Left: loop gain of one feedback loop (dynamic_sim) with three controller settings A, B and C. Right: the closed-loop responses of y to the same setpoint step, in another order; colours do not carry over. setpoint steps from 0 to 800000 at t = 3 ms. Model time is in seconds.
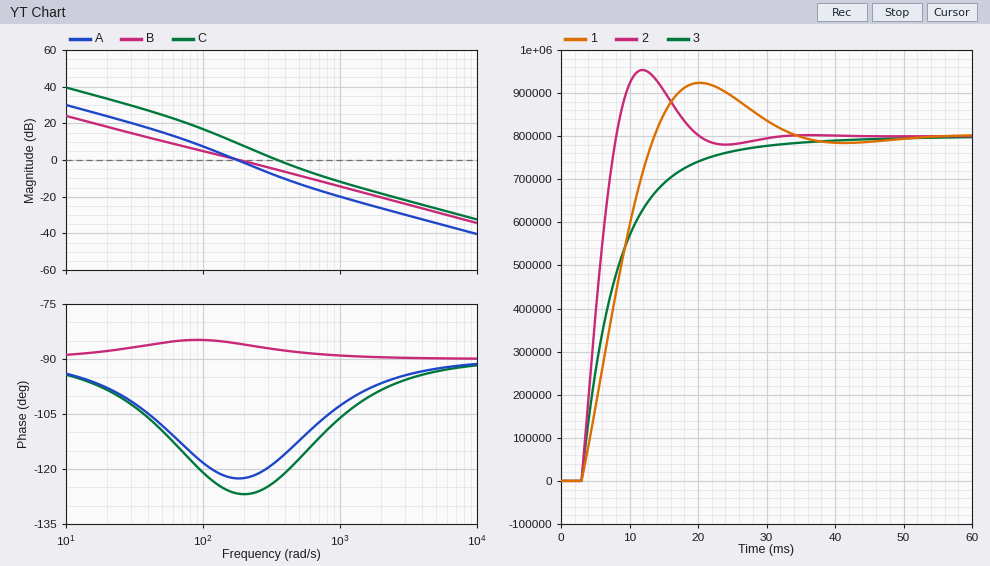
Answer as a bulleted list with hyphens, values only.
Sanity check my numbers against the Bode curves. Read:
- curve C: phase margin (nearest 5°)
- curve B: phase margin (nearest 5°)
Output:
- 55°
- 95°
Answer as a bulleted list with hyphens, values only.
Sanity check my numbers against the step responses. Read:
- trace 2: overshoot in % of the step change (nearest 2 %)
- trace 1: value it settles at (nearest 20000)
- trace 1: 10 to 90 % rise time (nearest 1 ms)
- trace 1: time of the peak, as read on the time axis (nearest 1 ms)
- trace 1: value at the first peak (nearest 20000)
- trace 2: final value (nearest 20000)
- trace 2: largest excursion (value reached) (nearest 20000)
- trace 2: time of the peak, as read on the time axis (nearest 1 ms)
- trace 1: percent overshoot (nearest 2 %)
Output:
- 20 %
- 800000
- 8 ms
- 20 ms
- 920000
- 800000
- 960000
- 12 ms
- 16 %
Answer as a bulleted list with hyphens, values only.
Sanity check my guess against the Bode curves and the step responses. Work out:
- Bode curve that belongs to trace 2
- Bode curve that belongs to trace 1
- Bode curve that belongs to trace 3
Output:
- C
- A
- B
